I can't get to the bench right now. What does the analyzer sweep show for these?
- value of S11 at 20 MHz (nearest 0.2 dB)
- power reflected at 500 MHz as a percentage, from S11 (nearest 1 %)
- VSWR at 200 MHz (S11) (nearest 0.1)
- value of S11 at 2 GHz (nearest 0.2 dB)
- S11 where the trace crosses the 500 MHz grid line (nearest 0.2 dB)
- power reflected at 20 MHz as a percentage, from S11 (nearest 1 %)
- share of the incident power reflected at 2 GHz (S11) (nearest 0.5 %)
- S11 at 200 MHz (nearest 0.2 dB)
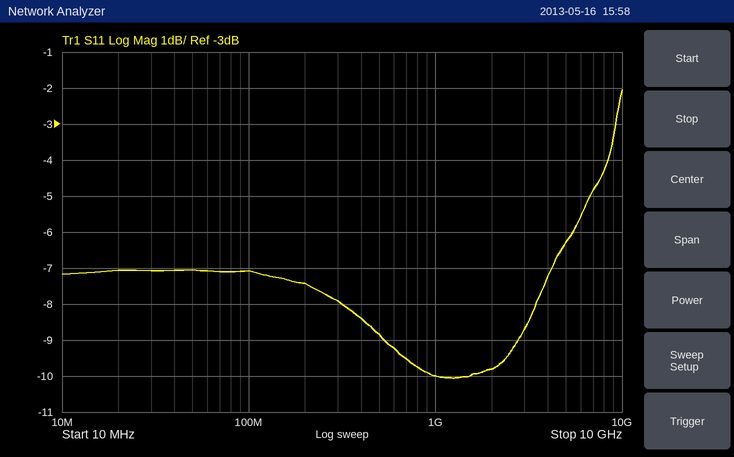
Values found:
-7.0 dB
13 %
2.5
-9.8 dB
-8.8 dB
20 %
10.5 %
-7.4 dB
